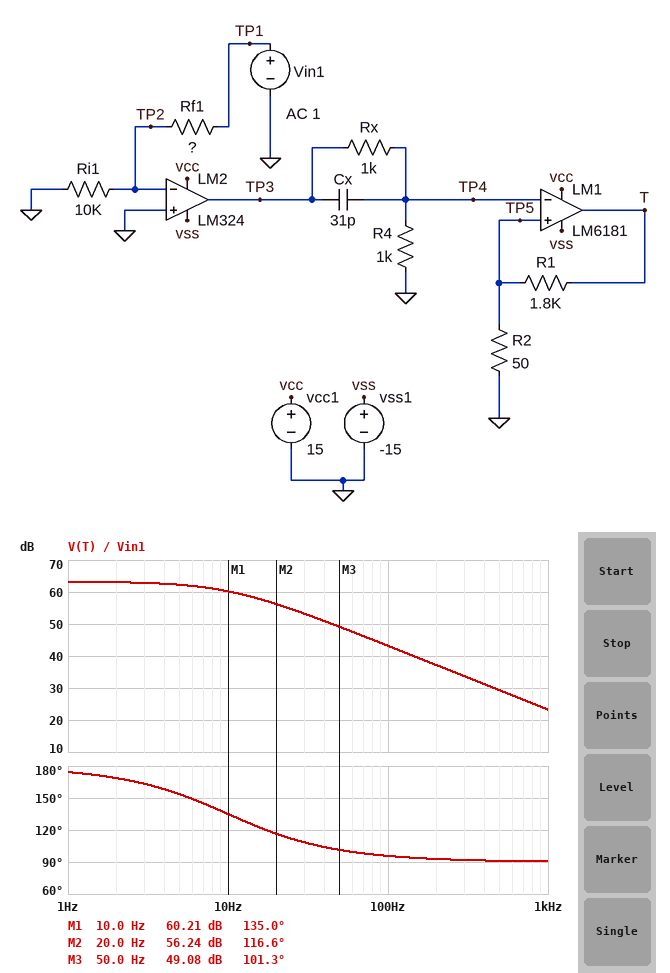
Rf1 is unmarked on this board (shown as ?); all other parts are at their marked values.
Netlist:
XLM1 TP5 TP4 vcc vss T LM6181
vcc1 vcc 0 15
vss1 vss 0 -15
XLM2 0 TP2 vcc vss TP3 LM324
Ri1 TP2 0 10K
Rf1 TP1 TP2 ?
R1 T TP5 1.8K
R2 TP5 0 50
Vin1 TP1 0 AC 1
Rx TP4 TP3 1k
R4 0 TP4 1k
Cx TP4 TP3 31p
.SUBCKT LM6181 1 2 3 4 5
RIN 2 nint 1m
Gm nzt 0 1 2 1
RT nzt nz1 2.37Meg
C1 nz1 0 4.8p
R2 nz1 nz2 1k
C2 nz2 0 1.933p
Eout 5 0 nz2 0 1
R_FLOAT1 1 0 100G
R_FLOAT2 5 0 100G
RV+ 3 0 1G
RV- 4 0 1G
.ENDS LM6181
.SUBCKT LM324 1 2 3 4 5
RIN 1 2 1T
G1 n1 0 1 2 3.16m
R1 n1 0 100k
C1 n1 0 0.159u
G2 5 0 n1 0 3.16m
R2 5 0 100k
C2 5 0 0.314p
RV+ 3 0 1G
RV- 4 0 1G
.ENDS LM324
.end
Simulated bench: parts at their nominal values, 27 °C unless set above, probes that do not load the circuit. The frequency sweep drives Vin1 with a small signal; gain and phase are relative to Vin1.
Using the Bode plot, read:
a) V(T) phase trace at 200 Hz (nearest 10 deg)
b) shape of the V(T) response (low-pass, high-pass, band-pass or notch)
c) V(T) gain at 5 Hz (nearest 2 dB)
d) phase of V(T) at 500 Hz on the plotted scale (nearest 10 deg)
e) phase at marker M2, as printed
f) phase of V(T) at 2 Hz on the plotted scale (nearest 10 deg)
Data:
90 deg
low-pass
62 dB
90 deg
116.6 deg
170 deg
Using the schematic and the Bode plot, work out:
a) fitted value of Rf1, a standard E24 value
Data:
240 kΩ
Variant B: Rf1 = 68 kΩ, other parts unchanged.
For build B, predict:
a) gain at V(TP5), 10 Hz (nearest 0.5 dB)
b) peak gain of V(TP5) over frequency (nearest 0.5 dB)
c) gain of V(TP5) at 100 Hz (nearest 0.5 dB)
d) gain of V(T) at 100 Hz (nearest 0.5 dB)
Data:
39.0 dB
42.0 dB
22.0 dB
53.5 dB
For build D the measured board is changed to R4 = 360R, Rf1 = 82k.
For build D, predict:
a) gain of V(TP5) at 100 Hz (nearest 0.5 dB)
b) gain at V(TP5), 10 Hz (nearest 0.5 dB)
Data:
11.5 dB
28.5 dB
